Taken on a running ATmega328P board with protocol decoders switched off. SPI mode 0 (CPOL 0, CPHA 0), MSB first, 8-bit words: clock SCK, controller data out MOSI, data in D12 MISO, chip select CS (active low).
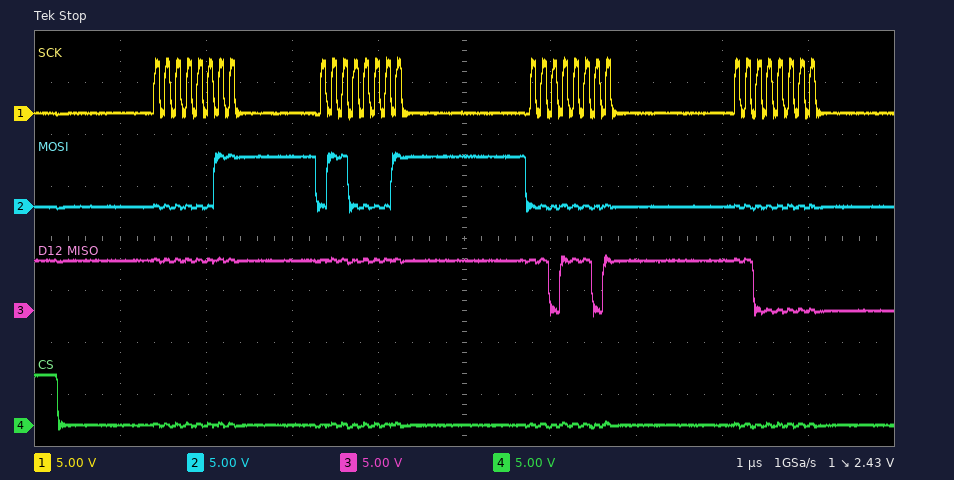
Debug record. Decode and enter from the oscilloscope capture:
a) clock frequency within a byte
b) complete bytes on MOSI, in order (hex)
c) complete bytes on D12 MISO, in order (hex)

8 MHz
03 61 00 00
FF FF DD C0
